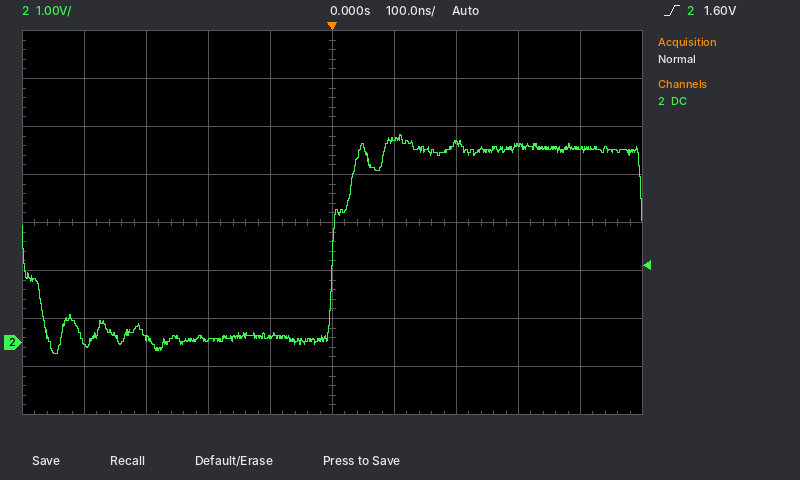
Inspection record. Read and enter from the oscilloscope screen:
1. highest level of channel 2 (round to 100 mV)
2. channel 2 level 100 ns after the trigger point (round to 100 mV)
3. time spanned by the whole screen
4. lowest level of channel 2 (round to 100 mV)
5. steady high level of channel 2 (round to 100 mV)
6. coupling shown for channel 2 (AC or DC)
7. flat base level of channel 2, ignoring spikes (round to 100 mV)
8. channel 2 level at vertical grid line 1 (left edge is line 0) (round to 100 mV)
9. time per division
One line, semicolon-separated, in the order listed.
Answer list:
4.3 V; 4.2 V; 1 µs; -200 mV; 4.0 V; DC; 100 mV; 0.0 V; 100 ns
